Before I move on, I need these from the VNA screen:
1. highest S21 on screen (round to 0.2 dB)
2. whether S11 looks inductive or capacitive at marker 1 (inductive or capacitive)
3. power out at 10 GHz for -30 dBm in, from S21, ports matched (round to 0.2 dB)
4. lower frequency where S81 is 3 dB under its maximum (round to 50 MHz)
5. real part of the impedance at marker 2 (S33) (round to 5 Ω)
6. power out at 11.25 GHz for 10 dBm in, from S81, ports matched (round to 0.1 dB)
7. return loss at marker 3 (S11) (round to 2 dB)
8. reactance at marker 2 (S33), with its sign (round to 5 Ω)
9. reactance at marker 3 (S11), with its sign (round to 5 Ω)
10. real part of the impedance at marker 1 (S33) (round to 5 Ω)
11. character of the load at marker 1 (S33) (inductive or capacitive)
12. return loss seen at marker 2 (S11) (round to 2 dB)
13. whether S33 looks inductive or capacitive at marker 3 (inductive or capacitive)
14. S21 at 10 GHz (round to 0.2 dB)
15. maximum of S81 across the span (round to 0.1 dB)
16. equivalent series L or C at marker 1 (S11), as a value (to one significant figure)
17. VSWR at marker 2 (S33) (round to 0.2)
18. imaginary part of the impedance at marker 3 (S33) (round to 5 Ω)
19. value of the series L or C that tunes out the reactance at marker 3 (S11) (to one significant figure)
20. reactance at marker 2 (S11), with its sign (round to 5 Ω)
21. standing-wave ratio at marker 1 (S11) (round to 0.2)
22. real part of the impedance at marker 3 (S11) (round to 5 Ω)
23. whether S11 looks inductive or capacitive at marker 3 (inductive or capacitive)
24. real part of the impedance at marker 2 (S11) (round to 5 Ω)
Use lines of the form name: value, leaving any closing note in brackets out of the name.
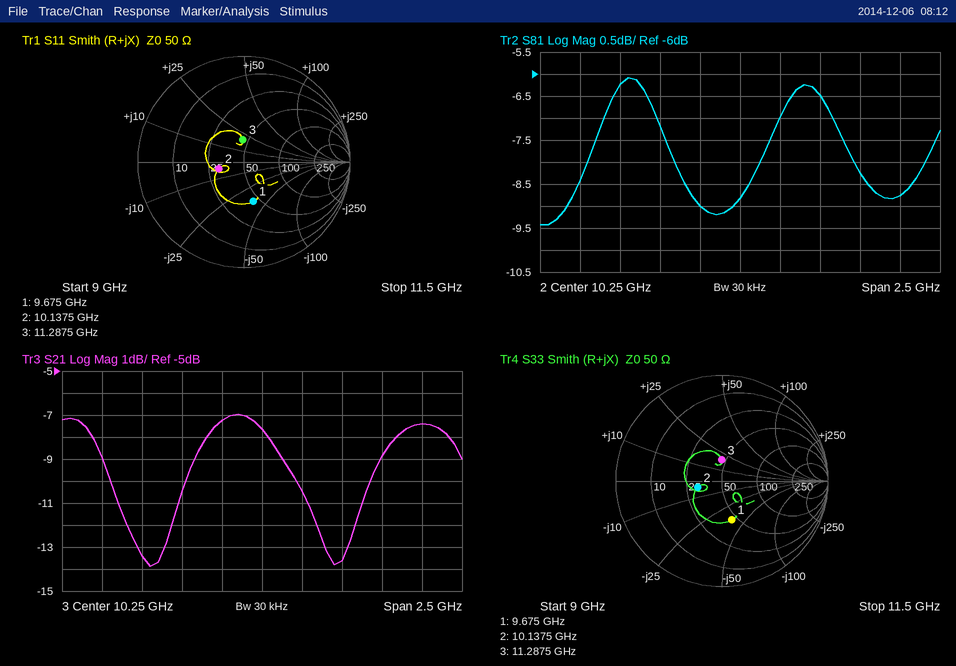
highest S21 on screen: -7.0 dB
whether S11 looks inductive or capacitive at marker 1: capacitive
power out at 10 GHz for -30 dBm in, from S21, ports matched: -37.2 dBm
lower frequency where S81 is 3 dB under its maximum: 9.15 GHz
real part of the impedance at marker 2 (S33): 30 Ω
power out at 11.25 GHz for 10 dBm in, from S81, ports matched: 1.2 dBm
return loss at marker 3 (S11): 14 dB
reactance at marker 2 (S33), with its sign: -5 Ω
reactance at marker 3 (S11), with its sign: +20 Ω
real part of the impedance at marker 1 (S33): 45 Ω
character of the load at marker 1 (S33): capacitive
return loss seen at marker 2 (S11): 12 dB
whether S33 looks inductive or capacitive at marker 3: inductive
S21 at 10 GHz: -7.2 dB
maximum of S81 across the span: -6.1 dB
equivalent series L or C at marker 1 (S11), as a value: 400 fF
VSWR at marker 2 (S33): 1.6
imaginary part of the impedance at marker 3 (S33): +20 Ω
value of the series L or C that tunes out the reactance at marker 3 (S11): 700 fF
reactance at marker 2 (S11), with its sign: -5 Ω
standing-wave ratio at marker 1 (S11): 2.2
real part of the impedance at marker 3 (S11): 45 Ω
whether S11 looks inductive or capacitive at marker 3: inductive
real part of the impedance at marker 2 (S11): 30 Ω
